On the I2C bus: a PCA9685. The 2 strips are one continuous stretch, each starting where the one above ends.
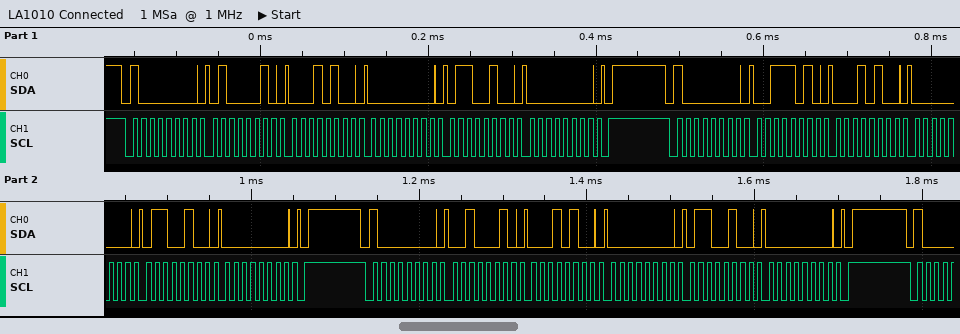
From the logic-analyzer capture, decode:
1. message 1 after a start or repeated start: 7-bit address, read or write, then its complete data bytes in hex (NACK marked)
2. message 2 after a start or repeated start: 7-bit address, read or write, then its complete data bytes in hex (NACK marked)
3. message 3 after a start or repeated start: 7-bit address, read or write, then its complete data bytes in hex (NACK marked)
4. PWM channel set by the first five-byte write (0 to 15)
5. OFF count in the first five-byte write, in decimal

0x40 write: 42 14 00 64 00
0x40 write: 3A 14 00 64 00
0x40 write: 22 14 00 64 00
15
100
